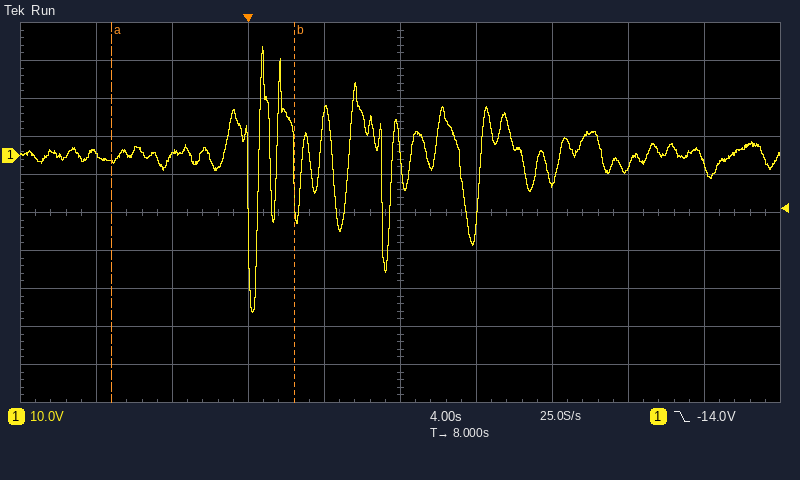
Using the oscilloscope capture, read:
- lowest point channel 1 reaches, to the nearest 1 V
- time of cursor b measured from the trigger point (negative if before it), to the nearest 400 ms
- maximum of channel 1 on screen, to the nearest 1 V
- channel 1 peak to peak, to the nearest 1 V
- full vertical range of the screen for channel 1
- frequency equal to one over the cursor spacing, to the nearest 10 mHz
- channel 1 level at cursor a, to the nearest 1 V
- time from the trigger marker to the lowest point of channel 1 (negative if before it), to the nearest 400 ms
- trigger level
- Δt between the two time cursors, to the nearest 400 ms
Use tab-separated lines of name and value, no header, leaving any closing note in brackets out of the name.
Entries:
lowest point channel 1 reaches, to the nearest 1 V	-41 V
time of cursor b measured from the trigger point (negative if before it), to the nearest 400 ms	+2.4 s
maximum of channel 1 on screen, to the nearest 1 V	29 V
channel 1 peak to peak, to the nearest 1 V	70 V
full vertical range of the screen for channel 1	100 V
frequency equal to one over the cursor spacing, to the nearest 10 mHz	100 mHz
channel 1 level at cursor a, to the nearest 1 V	-2 V
time from the trigger marker to the lowest point of channel 1 (negative if before it), to the nearest 400 ms	+400 ms
trigger level	-14.0 V
Δt between the two time cursors, to the nearest 400 ms	9.6 s
